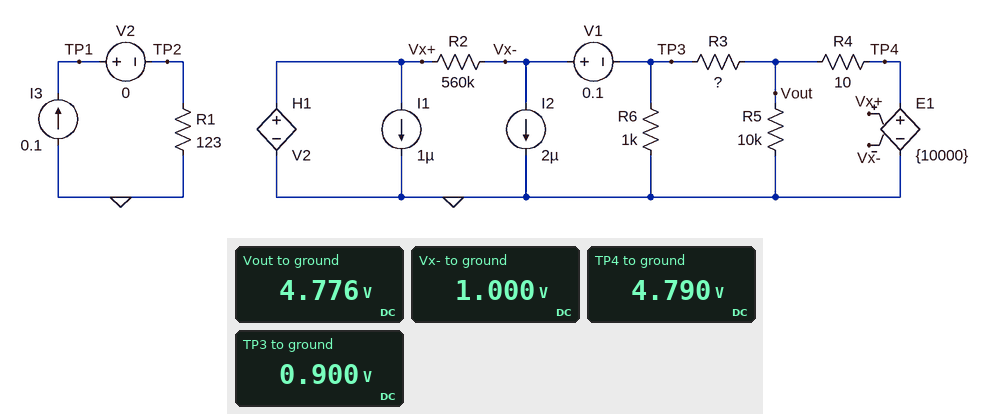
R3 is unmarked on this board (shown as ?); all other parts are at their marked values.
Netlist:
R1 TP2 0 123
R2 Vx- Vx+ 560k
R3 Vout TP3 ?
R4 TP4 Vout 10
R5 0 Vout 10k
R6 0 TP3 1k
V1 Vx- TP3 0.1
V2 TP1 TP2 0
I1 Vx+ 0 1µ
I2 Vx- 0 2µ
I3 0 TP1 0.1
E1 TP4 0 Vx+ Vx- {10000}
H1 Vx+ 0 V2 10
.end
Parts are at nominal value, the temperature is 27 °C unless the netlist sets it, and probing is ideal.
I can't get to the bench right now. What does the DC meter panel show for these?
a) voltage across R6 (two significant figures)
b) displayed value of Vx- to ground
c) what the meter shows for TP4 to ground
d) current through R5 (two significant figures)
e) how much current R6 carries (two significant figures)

900 mV
1.000 V
4.790 V
480 µA
900 µA
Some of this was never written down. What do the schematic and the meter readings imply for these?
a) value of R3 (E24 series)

4.3 kΩ
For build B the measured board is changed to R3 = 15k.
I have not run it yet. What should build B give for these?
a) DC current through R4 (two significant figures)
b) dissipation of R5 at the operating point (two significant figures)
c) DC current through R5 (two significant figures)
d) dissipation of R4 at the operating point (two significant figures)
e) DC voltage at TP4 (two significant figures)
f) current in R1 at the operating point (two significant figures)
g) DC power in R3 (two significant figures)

2.3 mA
21 mW
1.4 mA
55 µW
14 V
100 mA
12 mW
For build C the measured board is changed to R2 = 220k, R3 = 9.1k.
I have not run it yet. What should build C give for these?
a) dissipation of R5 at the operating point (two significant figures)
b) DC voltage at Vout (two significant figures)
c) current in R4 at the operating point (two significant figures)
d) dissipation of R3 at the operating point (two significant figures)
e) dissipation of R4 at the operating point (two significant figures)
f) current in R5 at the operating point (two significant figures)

8.3 mW
9.1 V
1.8 mA
7.4 mW
33 µW
910 µA
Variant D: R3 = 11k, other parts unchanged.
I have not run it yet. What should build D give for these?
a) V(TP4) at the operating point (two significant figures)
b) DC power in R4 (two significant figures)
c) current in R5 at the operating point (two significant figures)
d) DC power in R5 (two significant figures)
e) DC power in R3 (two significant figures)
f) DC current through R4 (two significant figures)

11 V
39 µW
1.1 mA
12 mW
8.9 mW
2.0 mA
